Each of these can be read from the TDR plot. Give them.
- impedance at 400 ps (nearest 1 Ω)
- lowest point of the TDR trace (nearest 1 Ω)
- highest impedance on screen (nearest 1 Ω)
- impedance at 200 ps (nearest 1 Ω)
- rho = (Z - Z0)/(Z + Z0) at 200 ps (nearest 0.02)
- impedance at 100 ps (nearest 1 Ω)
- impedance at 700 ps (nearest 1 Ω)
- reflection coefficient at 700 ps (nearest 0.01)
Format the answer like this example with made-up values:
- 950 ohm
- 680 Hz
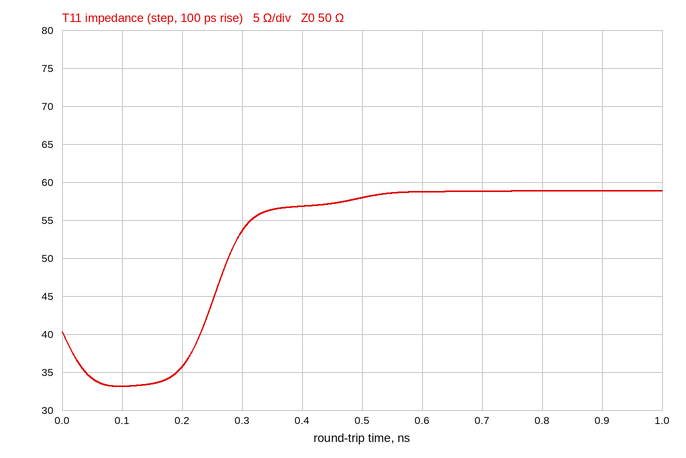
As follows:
- 57 Ω
- 33 Ω
- 59 Ω
- 36 Ω
- -0.16
- 33 Ω
- 59 Ω
- +0.08
